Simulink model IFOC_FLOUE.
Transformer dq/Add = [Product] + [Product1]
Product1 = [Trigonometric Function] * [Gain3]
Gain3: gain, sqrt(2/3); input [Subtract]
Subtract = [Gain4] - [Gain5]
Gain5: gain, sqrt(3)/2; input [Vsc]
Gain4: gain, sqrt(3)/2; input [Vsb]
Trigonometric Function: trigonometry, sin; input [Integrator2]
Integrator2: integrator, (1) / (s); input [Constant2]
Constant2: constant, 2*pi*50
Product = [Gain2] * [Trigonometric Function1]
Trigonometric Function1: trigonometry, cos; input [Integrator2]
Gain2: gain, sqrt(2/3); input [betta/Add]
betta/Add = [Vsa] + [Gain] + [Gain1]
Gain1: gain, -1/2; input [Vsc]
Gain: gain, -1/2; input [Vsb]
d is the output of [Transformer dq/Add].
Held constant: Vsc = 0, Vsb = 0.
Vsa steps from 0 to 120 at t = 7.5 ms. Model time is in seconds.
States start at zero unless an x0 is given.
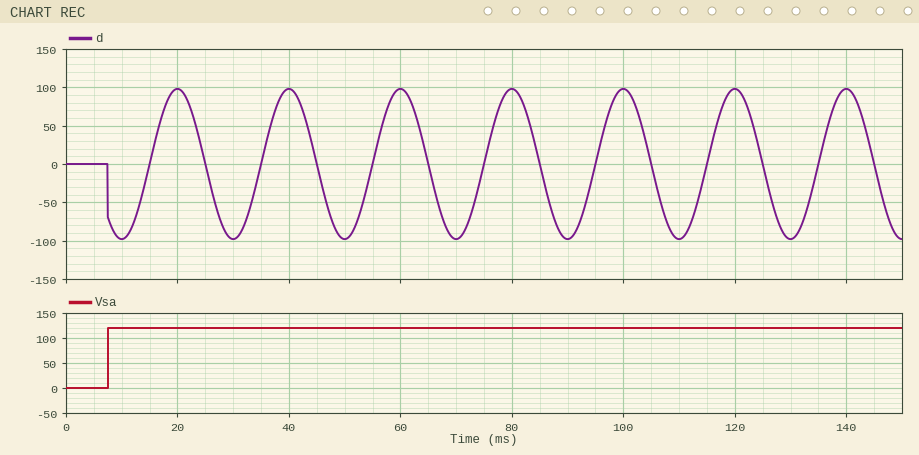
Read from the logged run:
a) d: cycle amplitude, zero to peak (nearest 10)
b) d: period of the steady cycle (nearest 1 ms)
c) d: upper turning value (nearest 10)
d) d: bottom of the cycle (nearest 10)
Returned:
100
20 ms
100
-100
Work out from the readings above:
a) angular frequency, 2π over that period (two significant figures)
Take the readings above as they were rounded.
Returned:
0.31 rad/ms
